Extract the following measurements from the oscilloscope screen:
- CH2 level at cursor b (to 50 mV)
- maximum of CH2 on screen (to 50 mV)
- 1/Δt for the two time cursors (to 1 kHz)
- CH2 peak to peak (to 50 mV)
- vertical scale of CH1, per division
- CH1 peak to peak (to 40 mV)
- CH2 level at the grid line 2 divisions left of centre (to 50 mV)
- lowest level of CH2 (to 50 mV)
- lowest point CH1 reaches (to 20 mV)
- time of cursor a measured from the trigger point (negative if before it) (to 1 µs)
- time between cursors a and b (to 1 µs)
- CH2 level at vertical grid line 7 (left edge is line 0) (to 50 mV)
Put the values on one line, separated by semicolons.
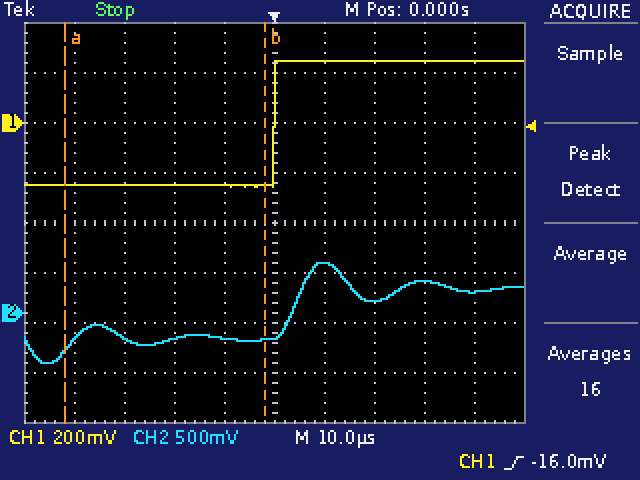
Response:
-250 mV; 500 mV; 25 kHz; 1.00 V; 200 mV; 520 mV; -250 mV; -500 mV; -260 mV; -42 µs; 40 µs; 100 mV
